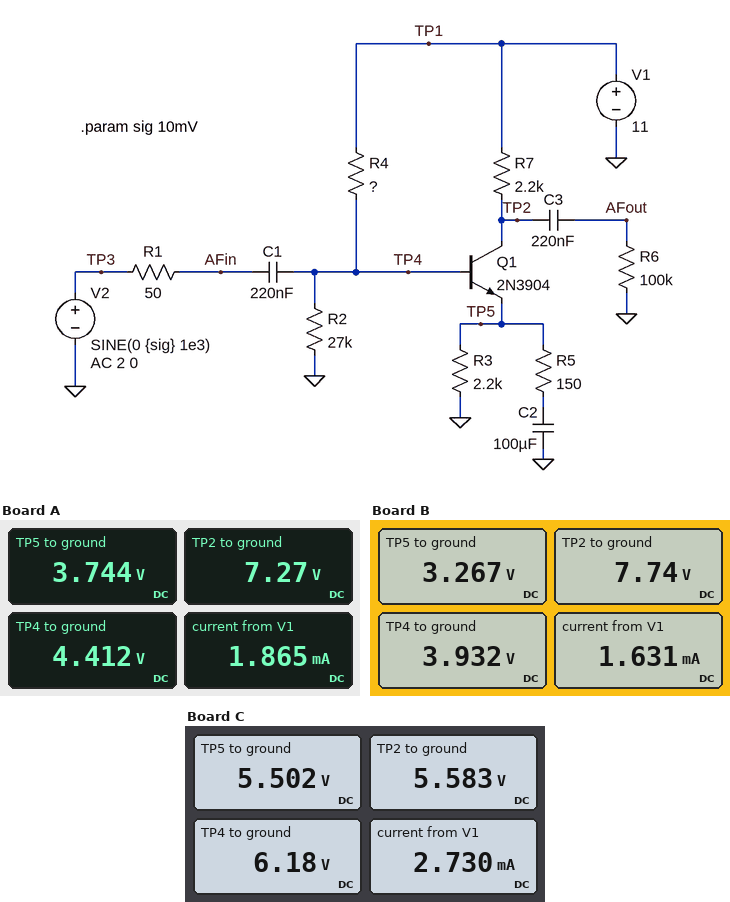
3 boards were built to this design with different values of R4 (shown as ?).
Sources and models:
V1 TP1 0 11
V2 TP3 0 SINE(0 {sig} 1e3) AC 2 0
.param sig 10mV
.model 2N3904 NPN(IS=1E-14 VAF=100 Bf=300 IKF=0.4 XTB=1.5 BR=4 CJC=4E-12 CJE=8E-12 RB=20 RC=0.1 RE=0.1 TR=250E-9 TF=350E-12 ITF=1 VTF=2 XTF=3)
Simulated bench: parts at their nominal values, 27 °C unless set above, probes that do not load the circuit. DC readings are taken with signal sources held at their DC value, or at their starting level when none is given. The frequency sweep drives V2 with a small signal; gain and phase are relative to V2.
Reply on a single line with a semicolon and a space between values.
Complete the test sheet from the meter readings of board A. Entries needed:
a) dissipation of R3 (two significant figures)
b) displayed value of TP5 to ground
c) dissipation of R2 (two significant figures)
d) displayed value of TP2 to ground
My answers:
6.4 mW; 3.744 V; 720 µW; 7.27 V
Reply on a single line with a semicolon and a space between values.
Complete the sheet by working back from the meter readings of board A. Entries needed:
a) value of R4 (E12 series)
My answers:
39 kΩ
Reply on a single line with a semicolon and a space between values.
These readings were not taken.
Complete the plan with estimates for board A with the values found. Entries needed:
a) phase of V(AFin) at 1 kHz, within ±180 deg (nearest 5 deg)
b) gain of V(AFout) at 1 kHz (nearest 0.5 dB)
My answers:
0 deg; 22.5 dB
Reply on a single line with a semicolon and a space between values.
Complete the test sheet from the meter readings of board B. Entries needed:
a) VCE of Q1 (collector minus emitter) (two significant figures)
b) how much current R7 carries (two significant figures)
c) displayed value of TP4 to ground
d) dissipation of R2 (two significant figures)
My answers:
4.5 V; 1.5 mA; 3.932 V; 570 µW
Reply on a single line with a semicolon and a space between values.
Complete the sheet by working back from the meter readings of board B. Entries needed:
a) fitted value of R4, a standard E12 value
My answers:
47 kΩ
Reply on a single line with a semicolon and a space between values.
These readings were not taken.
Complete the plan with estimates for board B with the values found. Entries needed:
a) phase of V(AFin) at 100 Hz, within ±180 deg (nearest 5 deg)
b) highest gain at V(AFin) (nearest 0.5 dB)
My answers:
0 deg; 0 dB
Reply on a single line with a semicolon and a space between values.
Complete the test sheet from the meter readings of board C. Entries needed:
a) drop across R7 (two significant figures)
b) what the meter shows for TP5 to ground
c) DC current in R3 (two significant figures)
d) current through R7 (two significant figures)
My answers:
5.4 V; 5.502 V; 2.5 mA; 2.5 mA
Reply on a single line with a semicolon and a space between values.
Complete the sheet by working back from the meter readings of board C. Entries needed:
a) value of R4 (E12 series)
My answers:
18 kΩ
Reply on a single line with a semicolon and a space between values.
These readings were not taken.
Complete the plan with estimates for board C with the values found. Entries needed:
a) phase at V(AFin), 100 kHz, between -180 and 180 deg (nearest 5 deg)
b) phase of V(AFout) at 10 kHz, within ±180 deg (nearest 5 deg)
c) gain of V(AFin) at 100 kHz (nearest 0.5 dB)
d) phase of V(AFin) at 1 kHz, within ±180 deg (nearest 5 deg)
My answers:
0 deg; -170 deg; -1.5 dB; -5 deg
